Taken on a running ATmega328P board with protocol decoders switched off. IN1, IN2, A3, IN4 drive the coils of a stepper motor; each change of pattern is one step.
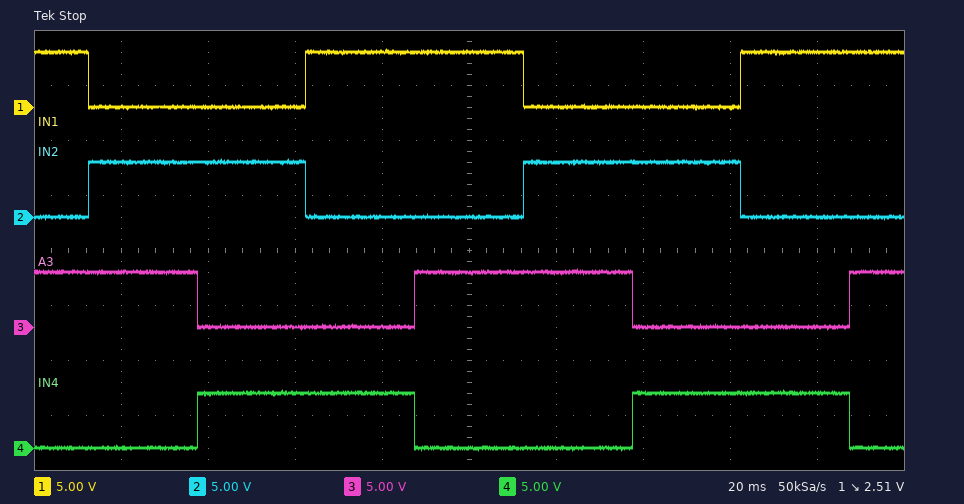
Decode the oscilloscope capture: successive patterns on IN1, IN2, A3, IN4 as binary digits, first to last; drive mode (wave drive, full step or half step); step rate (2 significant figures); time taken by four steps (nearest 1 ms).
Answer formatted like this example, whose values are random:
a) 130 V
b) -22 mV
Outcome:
a) 1010 0110 0101 1001 1010 0110 0101 1001 1010
b) full step
c) 40 steps/s
d) 100 ms
